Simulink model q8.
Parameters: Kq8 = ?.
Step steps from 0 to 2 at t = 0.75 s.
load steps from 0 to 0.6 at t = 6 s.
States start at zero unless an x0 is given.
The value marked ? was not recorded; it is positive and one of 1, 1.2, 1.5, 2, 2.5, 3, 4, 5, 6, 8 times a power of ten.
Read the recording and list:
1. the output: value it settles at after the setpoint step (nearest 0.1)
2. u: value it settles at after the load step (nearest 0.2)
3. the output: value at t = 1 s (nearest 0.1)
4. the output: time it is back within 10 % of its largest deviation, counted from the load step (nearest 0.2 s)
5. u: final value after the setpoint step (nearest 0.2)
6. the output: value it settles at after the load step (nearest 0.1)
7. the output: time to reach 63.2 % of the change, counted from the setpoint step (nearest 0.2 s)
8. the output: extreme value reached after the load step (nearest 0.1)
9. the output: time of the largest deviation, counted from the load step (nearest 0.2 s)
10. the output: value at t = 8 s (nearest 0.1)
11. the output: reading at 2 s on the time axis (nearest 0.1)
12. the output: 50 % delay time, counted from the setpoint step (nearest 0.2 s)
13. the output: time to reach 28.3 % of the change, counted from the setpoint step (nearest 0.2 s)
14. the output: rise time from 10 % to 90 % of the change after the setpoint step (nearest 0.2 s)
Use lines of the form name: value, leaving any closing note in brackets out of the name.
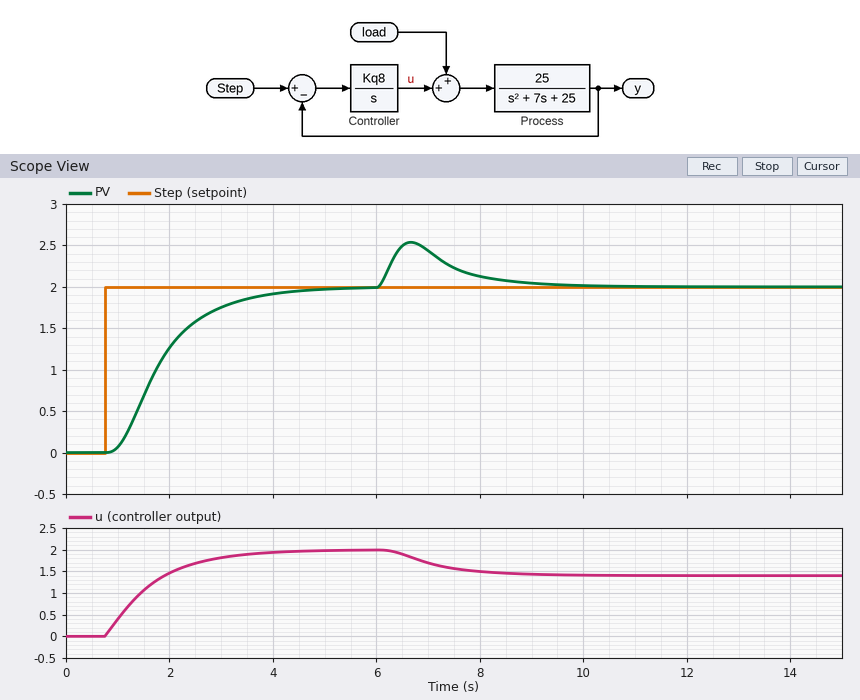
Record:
the output: value it settles at after the setpoint step: 2.0
u: value it settles at after the load step: 1.4
the output: value at t = 1 s: 0.1
the output: time it is back within 10 % of its largest deviation, counted from the load step: 2.8 s
u: final value after the setpoint step: 2.0
the output: value it settles at after the load step: 2.0
the output: time to reach 63.2 % of the change, counted from the setpoint step: 1.2 s
the output: extreme value reached after the load step: 2.5
the output: time of the largest deviation, counted from the load step: 0.6 s
the output: value at t = 8 s: 2.1
the output: reading at 2 s on the time axis: 1.3
the output: 50 % delay time, counted from the setpoint step: 1.0 s
the output: time to reach 28.3 % of the change, counted from the setpoint step: 0.6 s
the output: rise time from 10 % to 90 % of the change after the setpoint step: 2.0 s
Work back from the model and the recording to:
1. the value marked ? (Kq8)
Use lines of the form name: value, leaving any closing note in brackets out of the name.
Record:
the value marked ?: 0.8
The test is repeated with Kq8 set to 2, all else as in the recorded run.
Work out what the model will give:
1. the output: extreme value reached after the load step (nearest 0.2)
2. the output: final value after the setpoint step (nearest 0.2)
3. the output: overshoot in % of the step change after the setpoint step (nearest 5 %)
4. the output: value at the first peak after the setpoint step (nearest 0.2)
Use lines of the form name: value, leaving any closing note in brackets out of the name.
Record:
the output: extreme value reached after the load step: 2.4
the output: final value after the setpoint step: 2.0
the output: overshoot in % of the step change after the setpoint step: 15 %
the output: value at the first peak after the setpoint step: 2.2
